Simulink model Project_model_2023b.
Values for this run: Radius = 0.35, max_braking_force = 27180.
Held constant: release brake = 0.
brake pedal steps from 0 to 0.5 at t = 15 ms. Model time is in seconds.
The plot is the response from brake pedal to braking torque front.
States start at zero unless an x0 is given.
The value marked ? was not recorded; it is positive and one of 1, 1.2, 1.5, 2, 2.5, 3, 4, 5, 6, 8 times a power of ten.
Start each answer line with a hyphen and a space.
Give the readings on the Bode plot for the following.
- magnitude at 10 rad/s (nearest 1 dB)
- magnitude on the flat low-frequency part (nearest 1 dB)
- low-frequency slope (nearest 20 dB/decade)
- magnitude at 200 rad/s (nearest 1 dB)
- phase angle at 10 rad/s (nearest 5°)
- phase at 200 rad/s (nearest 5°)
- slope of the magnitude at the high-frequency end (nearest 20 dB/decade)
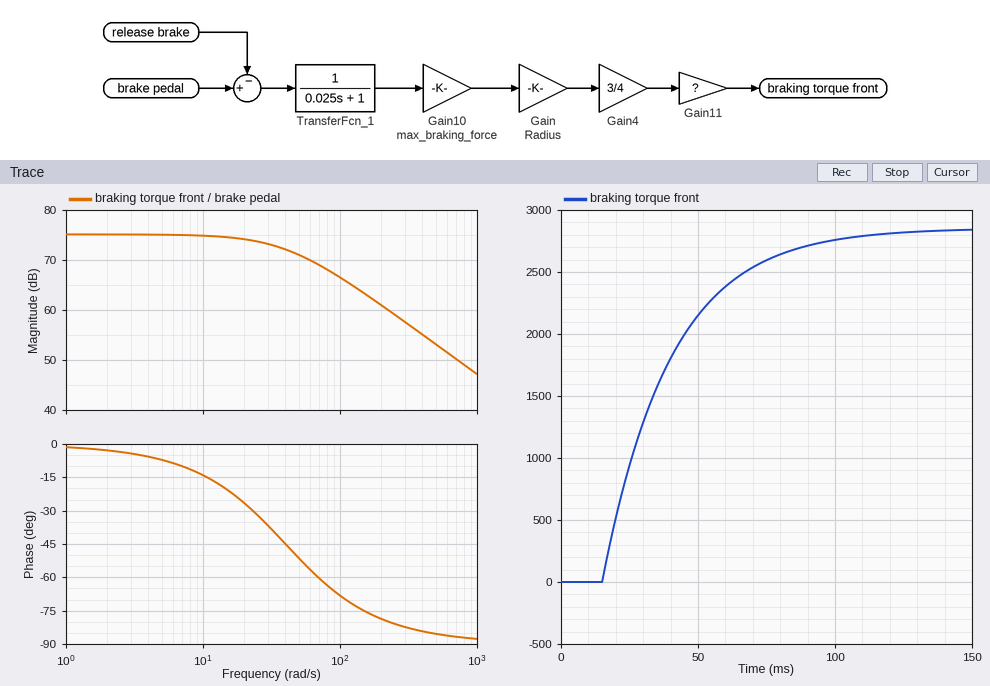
- 75 dB
- 75 dB
- 0 dB/decade
- 61 dB
- -15°
- -80°
- -20 dB/decade
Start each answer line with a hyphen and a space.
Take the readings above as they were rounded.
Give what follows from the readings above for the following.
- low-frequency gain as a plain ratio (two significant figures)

- 5600
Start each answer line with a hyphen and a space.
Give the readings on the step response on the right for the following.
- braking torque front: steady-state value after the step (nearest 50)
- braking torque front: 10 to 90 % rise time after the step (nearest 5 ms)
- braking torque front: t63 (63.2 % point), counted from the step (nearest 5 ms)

- 2850
- 55 ms
- 25 ms
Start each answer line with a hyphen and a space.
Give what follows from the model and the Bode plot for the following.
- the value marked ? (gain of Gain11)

- 0.8
